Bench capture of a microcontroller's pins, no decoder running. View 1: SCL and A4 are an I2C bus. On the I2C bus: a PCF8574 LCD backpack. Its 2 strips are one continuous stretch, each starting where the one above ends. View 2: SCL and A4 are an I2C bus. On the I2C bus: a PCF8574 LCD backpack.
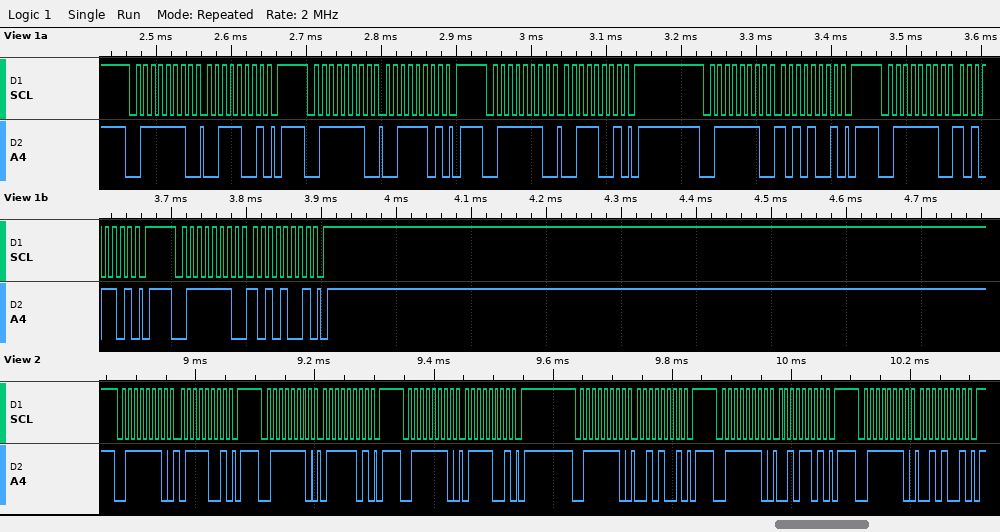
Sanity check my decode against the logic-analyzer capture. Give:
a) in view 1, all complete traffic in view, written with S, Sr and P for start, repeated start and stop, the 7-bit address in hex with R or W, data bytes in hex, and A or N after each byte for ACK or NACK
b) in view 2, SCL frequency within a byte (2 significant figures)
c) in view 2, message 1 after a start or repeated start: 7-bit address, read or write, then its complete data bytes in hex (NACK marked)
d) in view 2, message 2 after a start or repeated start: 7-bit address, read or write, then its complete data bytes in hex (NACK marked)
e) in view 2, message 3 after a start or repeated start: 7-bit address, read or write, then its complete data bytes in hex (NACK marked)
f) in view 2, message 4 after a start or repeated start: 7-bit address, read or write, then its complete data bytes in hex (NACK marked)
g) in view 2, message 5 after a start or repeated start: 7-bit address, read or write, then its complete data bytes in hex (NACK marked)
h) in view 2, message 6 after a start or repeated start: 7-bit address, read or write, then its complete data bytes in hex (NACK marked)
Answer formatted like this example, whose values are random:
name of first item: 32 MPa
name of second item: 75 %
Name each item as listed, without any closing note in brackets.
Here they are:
in view 1, all complete traffic in view, written with S, Sr and P for start, repeated start and stop, the 7-bit address in hex with R or W, data bytes in hex, and A or N after each byte for ACK or NACK: S 3FW A 39 A P S 3FW A 3D A P S 3FW A 39 A P S 3FW A A9 A P S 3FW A AD A P S 3FW A A9 A P
in view 2, SCL frequency within a byte: 100 kHz
in view 2, message 1 after a start or repeated start: 7-bit address, read or write, then its complete data bytes in hex: 0x3F write: 79
in view 2, message 2 after a start or repeated start: 7-bit address, read or write, then its complete data bytes in hex: 0x3F write: 7D
in view 2, message 3 after a start or repeated start: 7-bit address, read or write, then its complete data bytes in hex: 0x3F write: 79
in view 2, message 4 after a start or repeated start: 7-bit address, read or write, then its complete data bytes in hex: 0x3F write: 29
in view 2, message 5 after a start or repeated start: 7-bit address, read or write, then its complete data bytes in hex: 0x3F write: 2D
in view 2, message 6 after a start or repeated start: 7-bit address, read or write, then its complete data bytes in hex: 0x3F write: 29
